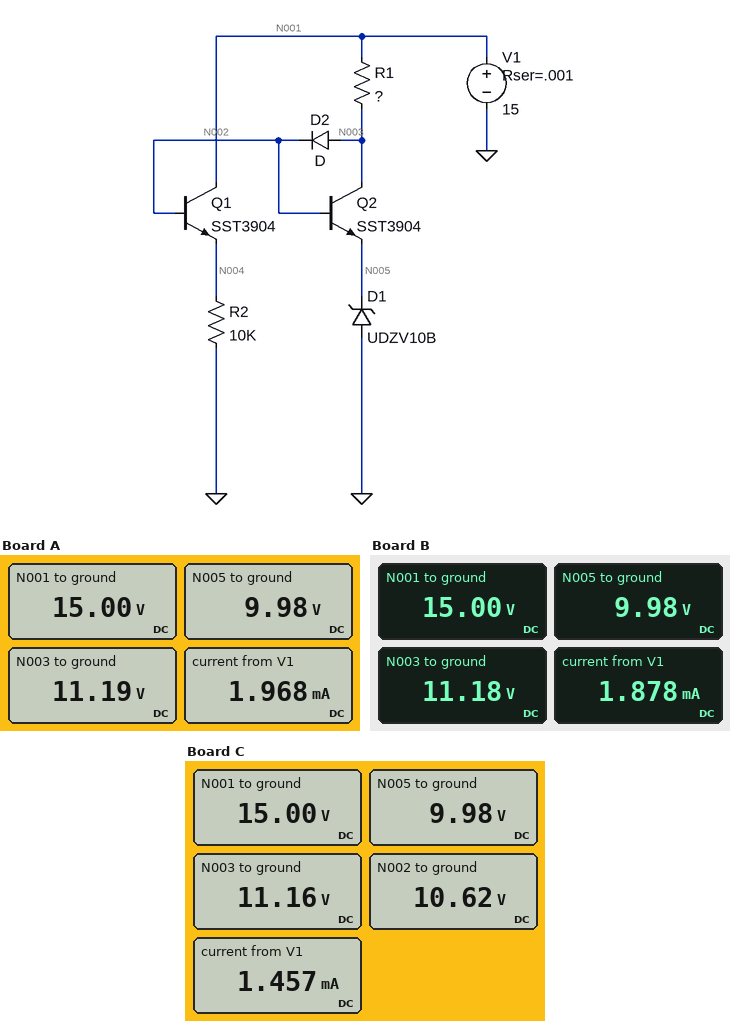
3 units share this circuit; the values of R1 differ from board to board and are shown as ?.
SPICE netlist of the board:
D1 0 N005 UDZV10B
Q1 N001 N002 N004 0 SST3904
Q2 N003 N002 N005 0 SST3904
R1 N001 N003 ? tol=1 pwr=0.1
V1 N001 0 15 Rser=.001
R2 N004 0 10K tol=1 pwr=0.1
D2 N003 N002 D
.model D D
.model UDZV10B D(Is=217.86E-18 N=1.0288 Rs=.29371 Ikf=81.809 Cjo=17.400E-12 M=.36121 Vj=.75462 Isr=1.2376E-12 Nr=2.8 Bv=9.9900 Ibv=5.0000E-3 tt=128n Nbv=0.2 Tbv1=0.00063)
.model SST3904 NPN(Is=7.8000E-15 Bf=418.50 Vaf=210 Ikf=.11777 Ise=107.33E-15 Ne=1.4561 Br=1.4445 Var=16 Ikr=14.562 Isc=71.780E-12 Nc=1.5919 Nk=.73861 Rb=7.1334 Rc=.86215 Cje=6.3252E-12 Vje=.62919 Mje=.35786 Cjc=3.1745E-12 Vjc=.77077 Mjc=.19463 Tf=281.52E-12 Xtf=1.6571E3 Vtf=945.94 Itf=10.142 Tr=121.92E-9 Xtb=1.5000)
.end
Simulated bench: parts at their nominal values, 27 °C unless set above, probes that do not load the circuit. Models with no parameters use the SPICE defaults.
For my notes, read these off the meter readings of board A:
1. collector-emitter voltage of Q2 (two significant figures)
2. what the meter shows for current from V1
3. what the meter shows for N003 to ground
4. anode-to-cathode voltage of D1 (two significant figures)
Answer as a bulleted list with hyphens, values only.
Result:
- 1.2 V
- 1.968 mA
- 11.19 V
- -10 V
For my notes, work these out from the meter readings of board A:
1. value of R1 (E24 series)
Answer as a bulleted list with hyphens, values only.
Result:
- 3.9 kΩ
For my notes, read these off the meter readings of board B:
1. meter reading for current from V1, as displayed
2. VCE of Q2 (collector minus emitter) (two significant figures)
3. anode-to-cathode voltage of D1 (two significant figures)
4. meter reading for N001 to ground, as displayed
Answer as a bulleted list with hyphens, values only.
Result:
- 1.878 mA
- 1.2 V
- -10 V
- 15.00 V
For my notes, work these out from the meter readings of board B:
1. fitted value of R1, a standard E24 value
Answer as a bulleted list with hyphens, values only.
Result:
- 4.3 kΩ
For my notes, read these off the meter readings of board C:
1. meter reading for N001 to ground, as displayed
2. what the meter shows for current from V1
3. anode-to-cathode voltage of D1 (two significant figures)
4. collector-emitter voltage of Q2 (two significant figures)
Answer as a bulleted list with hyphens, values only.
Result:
- 15.00 V
- 1.457 mA
- -10 V
- 1.2 V
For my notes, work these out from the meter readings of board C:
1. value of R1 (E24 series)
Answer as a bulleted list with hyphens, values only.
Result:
- 8.2 kΩ
